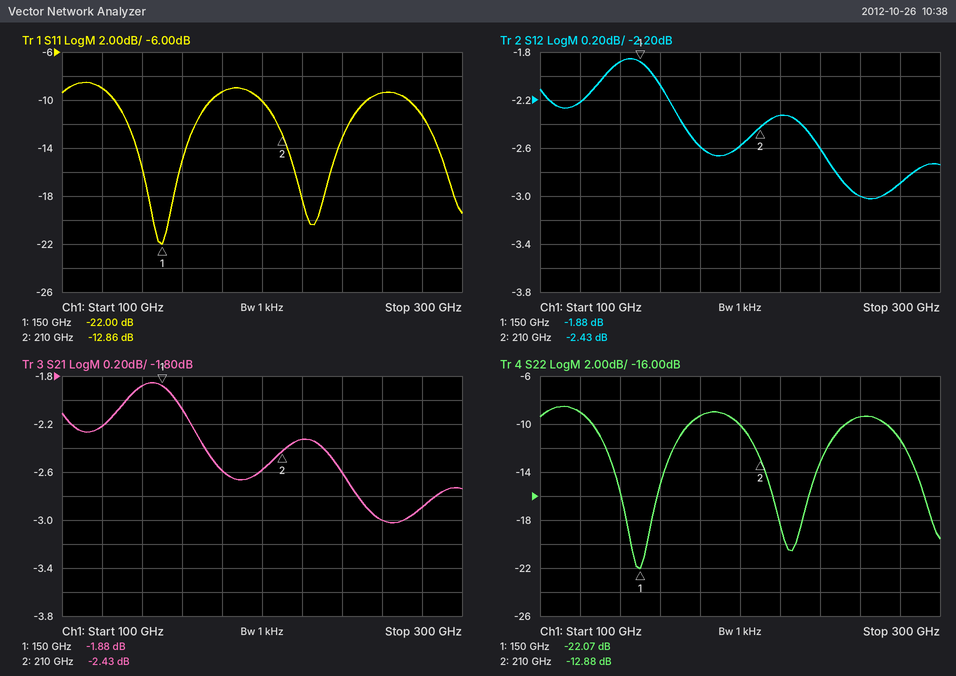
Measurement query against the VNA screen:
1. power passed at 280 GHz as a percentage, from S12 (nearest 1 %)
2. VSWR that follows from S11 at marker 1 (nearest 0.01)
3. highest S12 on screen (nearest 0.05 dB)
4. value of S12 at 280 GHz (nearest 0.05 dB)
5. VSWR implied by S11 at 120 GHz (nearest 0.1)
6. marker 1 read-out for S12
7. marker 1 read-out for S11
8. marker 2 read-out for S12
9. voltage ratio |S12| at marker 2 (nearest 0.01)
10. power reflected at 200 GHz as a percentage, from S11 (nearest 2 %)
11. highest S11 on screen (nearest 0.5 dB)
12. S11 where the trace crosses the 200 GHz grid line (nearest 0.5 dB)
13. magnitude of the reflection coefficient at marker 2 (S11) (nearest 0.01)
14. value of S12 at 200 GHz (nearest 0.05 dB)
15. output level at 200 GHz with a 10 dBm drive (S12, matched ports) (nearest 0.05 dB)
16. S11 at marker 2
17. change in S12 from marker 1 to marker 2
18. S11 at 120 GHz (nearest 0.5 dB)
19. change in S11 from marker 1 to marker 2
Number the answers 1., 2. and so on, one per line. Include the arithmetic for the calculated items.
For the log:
1. 10^(-2.9/10) ≈ 51 %
2. (1 + 0.0794)/(1 − 0.0794) ≈ 1.17
3. -1.85 dB
4. -2.90 dB
5. |Γ| = 10^(-9/20) = 0.3548; VSWR = (1 + 0.3548)/(1 − 0.3548) ≈ 2.1
6. -1.88 dB
7. -22.00 dB
8. -2.43 dB
9. 10^(-2.43/20) ≈ 0.76
10. 10^(-10/10) ≈ 10 %
11. -8.5 dB
12. -10.0 dB
13. 10^(-12.86/20) ≈ 0.23
14. -2.60 dB
15. 10 dBm + (-2.60 dB) = 7.40 dBm
16. -12.86 dB
17. -2.43 − (-1.88) = -0.55 dB
18. -9.0 dB
19. -12.86 − (-22) = 9.14 dB
